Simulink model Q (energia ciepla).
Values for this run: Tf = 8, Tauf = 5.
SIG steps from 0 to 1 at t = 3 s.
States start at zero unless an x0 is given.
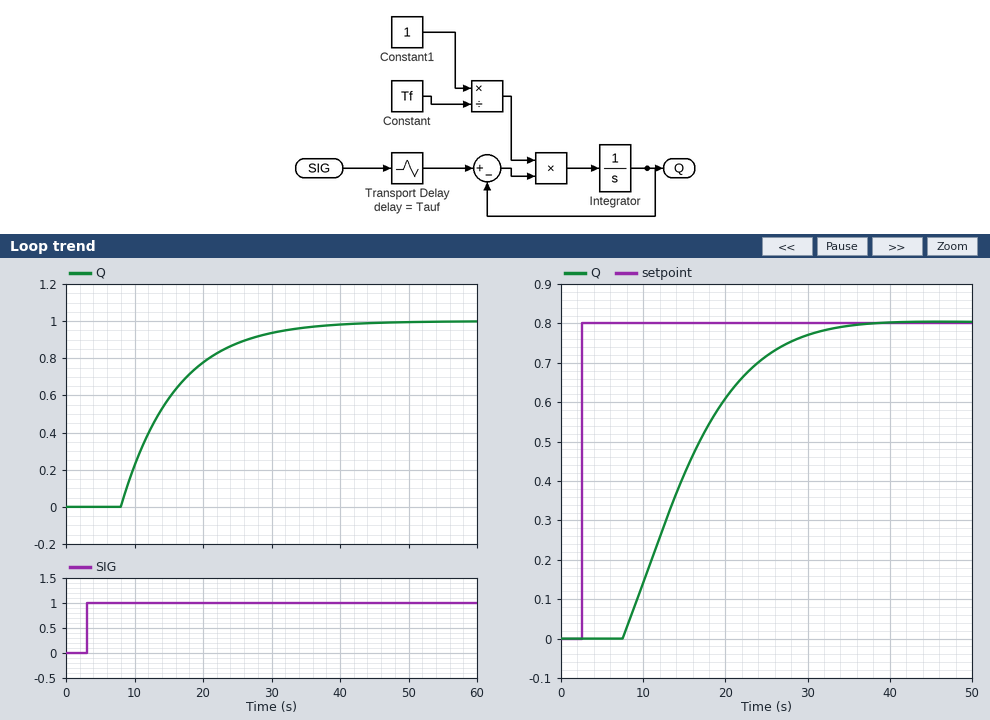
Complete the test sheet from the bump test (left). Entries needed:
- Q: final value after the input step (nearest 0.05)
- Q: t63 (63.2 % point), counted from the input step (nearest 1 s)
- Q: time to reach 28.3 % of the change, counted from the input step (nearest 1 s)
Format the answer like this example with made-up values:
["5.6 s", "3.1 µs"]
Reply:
["1.00", "13 s", "8 s"]
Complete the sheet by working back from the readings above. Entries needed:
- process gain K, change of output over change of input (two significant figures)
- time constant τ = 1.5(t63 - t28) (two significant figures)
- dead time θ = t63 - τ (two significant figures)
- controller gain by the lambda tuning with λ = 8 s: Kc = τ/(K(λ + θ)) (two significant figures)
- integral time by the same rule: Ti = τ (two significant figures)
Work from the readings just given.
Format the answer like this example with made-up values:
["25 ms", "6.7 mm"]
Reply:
["1.0", "7.5 s", "5.5 s", "0.56", "7.5 s"]
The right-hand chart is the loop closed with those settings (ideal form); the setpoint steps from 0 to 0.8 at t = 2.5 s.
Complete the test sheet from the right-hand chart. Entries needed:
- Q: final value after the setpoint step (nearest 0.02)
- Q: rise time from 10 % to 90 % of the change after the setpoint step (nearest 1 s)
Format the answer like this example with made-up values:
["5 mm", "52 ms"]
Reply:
["0.80", "16 s"]
